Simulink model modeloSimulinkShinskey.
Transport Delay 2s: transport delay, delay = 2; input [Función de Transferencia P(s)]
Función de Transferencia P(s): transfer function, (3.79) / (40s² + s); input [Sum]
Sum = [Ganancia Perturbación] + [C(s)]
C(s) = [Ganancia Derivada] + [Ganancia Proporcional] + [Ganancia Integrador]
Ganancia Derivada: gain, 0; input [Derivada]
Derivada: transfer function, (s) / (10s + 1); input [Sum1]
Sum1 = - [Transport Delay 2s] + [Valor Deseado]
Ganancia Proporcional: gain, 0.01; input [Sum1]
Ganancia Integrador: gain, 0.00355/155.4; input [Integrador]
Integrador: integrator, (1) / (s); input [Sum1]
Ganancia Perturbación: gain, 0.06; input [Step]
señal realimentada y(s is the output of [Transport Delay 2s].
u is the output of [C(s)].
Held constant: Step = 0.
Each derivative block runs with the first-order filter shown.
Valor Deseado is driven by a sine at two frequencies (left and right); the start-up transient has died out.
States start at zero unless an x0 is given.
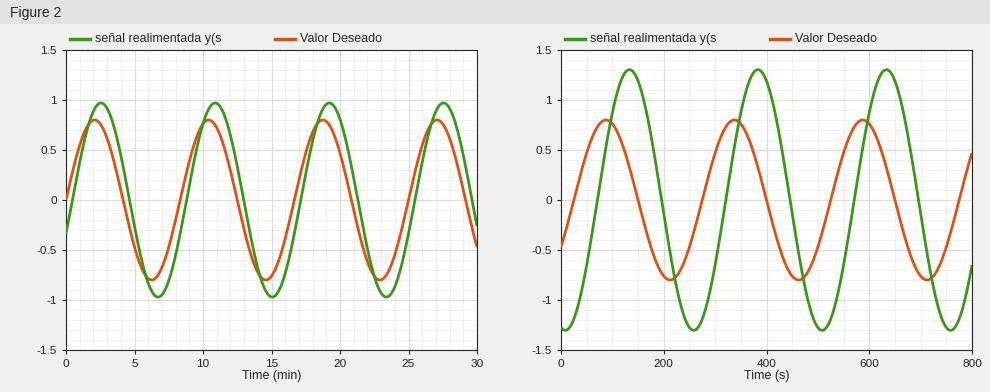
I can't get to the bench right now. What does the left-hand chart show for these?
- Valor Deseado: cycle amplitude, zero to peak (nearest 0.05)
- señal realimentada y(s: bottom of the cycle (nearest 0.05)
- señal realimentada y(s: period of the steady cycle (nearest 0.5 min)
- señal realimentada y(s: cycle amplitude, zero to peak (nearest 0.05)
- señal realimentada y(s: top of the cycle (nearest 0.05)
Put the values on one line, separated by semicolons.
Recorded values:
0.80; -0.95; 8.5 min; 0.95; 0.95
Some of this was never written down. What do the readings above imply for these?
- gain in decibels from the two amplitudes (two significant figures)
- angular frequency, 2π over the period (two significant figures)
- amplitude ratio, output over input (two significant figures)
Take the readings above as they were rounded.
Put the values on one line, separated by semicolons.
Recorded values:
1.5 dB; 0.74 rad/min; 1.2
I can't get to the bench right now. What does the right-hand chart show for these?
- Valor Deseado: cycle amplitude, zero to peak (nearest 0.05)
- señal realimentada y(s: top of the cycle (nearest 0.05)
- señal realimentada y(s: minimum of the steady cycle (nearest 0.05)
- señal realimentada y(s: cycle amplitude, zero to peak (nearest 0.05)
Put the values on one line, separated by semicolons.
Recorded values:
0.80; 1.30; -1.30; 1.30
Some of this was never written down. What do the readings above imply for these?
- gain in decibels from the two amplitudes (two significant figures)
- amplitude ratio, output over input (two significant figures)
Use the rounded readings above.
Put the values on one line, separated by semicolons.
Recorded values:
4.2 dB; 1.6
